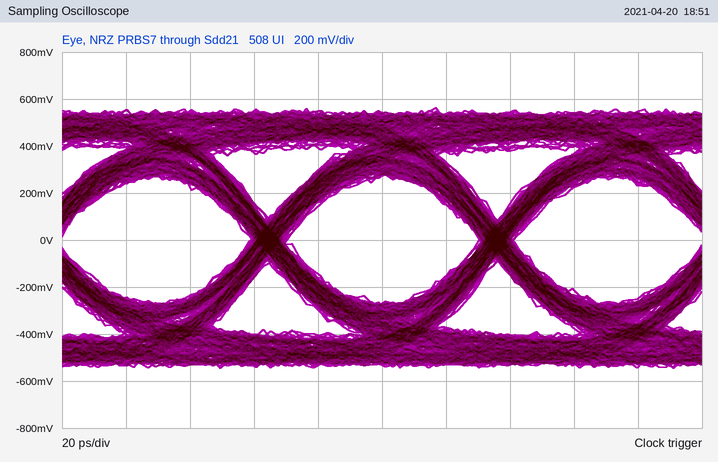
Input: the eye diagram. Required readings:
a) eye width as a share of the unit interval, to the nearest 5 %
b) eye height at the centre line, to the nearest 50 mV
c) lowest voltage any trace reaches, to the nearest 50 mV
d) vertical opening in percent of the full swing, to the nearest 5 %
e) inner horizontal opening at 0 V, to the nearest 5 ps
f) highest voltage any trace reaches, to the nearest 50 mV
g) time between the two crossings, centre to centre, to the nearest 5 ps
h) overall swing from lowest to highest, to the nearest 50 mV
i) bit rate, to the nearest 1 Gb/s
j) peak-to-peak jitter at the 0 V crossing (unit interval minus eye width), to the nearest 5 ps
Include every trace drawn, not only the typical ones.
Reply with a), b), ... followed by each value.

a) 85 %
b) 550 mV
c) -550 mV
d) 50 %
e) 60 ps
f) 550 mV
g) 70 ps
h) 1.10 V
i) 14 Gb/s
j) 10 ps
